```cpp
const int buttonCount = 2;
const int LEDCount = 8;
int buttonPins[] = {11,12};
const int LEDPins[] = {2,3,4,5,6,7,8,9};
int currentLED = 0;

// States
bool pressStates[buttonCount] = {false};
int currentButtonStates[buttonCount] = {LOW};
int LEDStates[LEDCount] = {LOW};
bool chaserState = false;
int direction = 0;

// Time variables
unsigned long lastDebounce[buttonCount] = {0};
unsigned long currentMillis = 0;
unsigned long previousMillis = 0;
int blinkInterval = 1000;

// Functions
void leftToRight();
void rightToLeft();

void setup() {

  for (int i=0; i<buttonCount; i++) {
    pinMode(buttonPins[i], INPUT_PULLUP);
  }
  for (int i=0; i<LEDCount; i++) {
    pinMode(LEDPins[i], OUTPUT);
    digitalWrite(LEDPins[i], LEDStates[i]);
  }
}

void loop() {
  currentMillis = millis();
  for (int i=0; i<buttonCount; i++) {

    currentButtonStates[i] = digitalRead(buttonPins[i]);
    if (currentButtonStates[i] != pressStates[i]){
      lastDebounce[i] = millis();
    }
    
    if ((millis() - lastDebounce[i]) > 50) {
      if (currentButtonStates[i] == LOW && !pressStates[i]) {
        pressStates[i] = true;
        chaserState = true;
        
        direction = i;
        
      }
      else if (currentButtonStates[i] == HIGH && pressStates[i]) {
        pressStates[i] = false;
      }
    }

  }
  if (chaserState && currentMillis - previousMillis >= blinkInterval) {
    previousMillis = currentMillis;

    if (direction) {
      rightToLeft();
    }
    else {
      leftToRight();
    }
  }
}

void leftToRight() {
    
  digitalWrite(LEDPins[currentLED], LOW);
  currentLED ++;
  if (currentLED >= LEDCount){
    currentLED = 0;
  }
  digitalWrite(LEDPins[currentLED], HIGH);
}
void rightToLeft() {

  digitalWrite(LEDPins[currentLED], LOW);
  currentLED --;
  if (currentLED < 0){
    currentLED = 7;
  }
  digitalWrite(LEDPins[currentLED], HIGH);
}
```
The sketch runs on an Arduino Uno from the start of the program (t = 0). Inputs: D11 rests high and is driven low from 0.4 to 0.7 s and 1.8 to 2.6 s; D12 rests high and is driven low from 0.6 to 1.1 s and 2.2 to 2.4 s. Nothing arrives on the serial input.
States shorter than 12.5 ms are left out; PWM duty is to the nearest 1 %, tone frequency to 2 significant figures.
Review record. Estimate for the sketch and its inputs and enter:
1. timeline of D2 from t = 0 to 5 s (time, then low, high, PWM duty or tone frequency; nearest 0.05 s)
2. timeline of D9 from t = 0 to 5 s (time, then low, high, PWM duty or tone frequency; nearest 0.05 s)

0 s low; 2 s high; 3 s low
0 s low; 1 s high; 2 s low; 3 s high; 4 s low
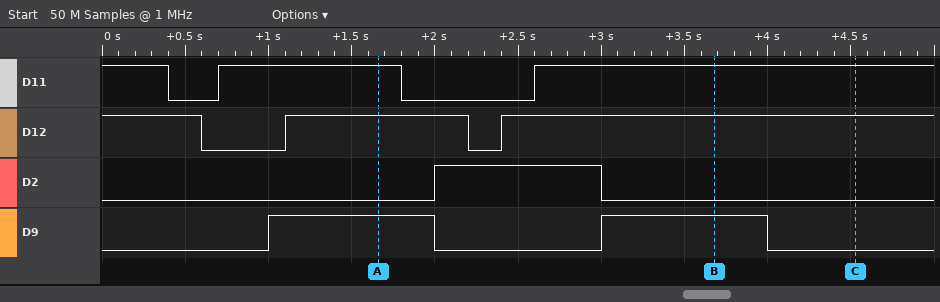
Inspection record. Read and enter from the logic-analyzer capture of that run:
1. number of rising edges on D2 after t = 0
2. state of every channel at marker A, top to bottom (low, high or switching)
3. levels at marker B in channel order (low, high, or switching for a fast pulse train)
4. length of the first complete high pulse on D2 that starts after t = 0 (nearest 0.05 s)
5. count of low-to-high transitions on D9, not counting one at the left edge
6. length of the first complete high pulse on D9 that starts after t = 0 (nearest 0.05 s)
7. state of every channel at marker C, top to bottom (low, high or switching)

1
D11 high, D12 high, D2 low, D9 high
D11 high, D12 high, D2 low, D9 high
1.00 s
2
1.00 s
D11 high, D12 high, D2 low, D9 low
